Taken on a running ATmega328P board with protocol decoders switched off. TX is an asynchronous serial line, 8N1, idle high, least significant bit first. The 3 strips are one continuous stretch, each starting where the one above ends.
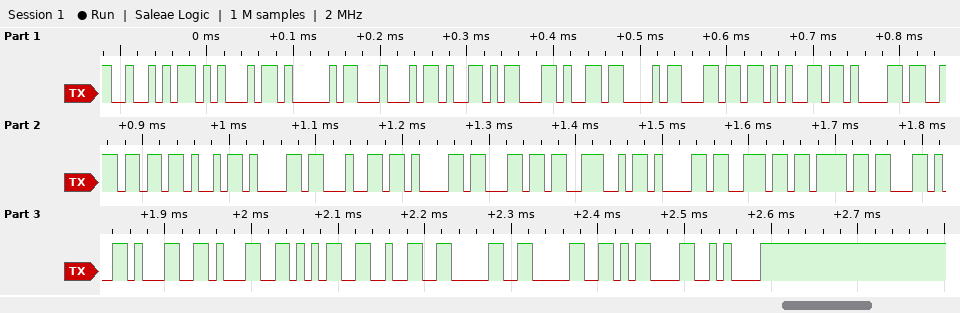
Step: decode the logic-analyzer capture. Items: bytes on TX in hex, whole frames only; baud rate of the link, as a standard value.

52 45 41 44 59 2C 43 6C 65 61 6E 4B 61 64 61 6C 4E 61 6E 6F 2C 31 31 35 32 30 30 0D 0A
115200 baud
